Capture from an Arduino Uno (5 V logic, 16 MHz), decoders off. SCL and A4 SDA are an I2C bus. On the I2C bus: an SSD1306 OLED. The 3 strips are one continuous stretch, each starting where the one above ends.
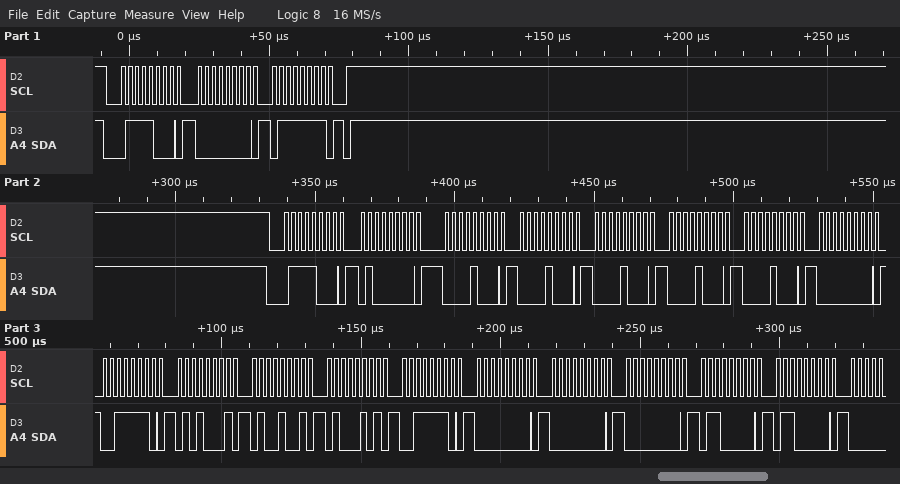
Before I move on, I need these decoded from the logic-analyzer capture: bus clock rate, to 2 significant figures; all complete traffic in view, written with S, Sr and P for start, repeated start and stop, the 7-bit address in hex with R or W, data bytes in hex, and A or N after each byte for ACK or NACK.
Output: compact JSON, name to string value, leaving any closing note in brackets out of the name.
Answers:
{"bus clock rate, to 2 significant figures": "400 kHz", "all complete traffic in view, written with S, Sr and P for start, repeated start and stop, the 7-bit address in hex with R or W, data bytes in hex, and A or N after each byte for ACK or NACK": "S 3CW A 00 A 7F A P S 3CW A 40 A 08 A 08 A 08 A 08 A 08 A 00 A 3E A 51 A 49 A 45 A 3E A 00 A 00 A 00 A 60 A 60 A"}
